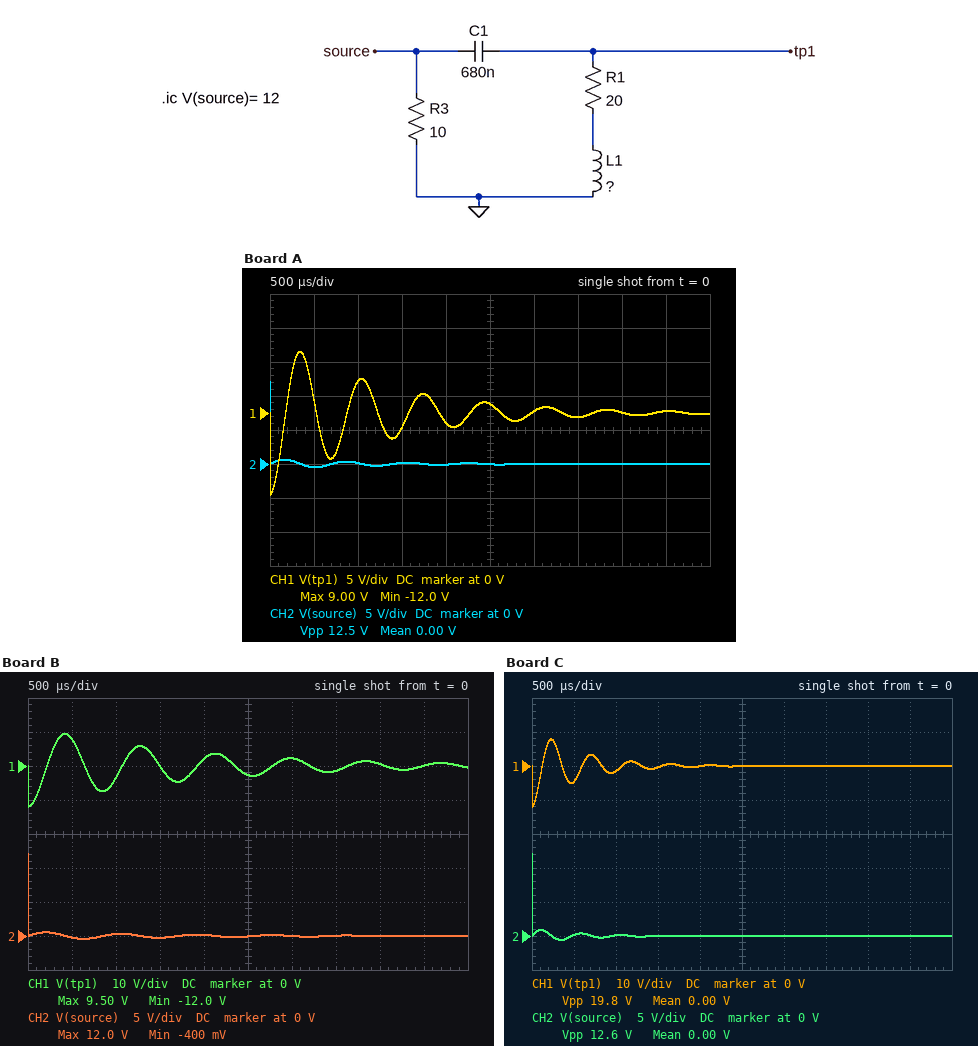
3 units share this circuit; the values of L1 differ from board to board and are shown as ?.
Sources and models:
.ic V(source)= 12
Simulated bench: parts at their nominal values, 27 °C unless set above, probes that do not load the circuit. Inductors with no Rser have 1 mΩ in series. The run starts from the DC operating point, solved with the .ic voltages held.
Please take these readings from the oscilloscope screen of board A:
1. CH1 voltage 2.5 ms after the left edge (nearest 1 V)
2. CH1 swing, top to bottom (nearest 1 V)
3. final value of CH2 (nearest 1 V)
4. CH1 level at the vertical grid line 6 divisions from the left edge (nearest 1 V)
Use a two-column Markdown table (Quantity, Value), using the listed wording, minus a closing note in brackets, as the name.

| Quantity | Value |
|---|---|
| CH1 voltage 2.5 ms after the left edge | 1 V |
| CH1 swing, top to bottom | 21 V |
| final value of CH2 | 0 V |
| CH1 level at the vertical grid line 6 divisions from the left edge | 0 V |
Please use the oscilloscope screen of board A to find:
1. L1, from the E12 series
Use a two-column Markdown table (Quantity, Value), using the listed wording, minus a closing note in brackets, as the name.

| Quantity | Value |
|---|---|
| L1, from the E12 series | 18 mH |
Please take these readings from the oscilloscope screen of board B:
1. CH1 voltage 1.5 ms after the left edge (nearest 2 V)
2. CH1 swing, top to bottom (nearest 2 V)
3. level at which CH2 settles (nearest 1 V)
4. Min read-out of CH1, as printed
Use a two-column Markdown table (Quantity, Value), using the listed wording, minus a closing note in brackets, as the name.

| Quantity | Value |
|---|---|
| CH1 voltage 1.5 ms after the left edge | 0 V |
| CH1 swing, top to bottom | 22 V |
| level at which CH2 settles | 0 V |
| Min read-out of CH1, as printed | -12.0 V |
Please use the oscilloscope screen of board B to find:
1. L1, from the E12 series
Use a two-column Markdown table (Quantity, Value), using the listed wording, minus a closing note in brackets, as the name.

| Quantity | Value |
|---|---|
| L1, from the E12 series | 27 mH |
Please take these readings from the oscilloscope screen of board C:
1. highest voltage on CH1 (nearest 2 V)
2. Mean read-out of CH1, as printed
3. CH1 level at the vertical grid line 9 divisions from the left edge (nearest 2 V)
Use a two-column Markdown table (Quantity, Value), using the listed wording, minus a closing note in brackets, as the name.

| Quantity | Value |
|---|---|
| highest voltage on CH1 | 8 V |
| Mean read-out of CH1, as printed | 0.00 V |
| CH1 level at the vertical grid line 9 divisions from the left edge | 0 V |
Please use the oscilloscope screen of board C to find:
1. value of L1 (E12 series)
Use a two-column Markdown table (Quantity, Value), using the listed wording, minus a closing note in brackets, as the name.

| Quantity | Value |
|---|---|
| value of L1 | 8.2 mH |
